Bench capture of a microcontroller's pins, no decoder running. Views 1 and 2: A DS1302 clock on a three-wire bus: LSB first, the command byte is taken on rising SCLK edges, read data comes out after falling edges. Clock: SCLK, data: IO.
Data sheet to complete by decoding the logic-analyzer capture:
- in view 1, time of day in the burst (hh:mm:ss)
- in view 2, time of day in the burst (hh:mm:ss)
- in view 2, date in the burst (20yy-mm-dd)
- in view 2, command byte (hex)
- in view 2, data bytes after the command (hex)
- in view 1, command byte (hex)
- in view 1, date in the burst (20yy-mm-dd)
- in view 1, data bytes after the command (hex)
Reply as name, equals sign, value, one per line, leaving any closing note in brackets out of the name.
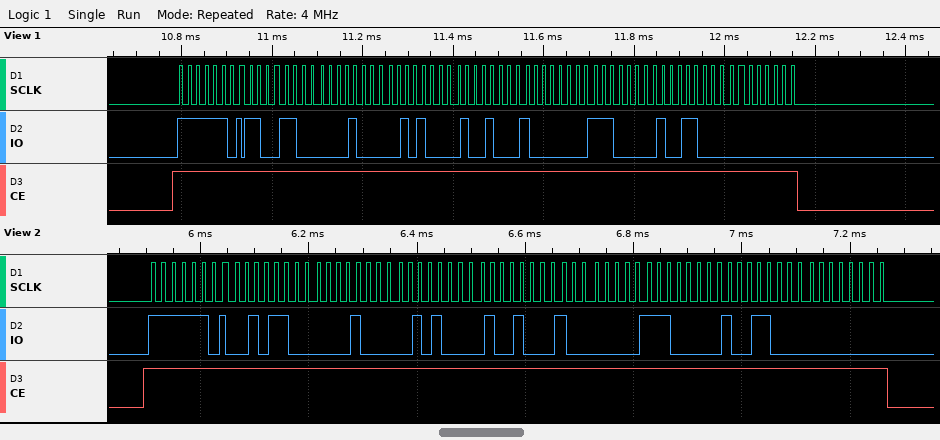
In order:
in view 1, time of day in the burst = 14:10:33
in view 2, time of day in the burst = 14:10:34
in view 2, date in the burst = 2019-01-12
in view 2, command byte = 0xBF
in view 2, data bytes after the command = 34 10 14 12 01 07 19 00
in view 1, command byte = 0xBF
in view 1, date in the burst = 2019-01-12
in view 1, data bytes after the command = 33 10 14 12 01 07 19 00
